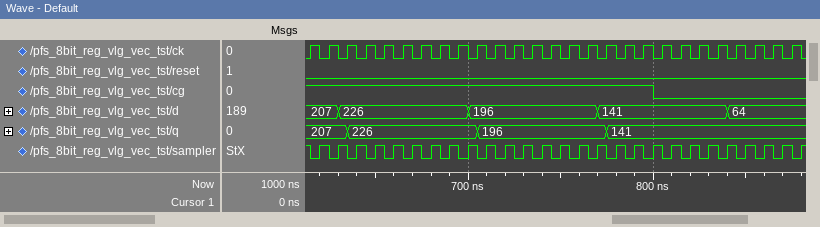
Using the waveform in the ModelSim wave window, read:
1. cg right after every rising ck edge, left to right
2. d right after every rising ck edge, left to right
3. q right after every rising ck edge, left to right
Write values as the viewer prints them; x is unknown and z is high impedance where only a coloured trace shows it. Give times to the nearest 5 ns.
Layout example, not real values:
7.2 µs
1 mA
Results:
1 1 1 1 1 1 1 1 1 1 1 1 1 1 1 1 1 1 1 0 0 0 0 0 0 0 0
207, 207, 226, 226, 226, 226, 226, 226, 226, 196, 196, 196, 196, 196, 196, 196, 141, 141, 141, 141, 141, 141, 141, 64, 64, 64, 64
207, 207, 226, 226, 226, 226, 226, 226, 226, 196, 196, 196, 196, 196, 196, 196, 141, 141, 141, 141, 141, 141, 141, 141, 141, 141, 141
